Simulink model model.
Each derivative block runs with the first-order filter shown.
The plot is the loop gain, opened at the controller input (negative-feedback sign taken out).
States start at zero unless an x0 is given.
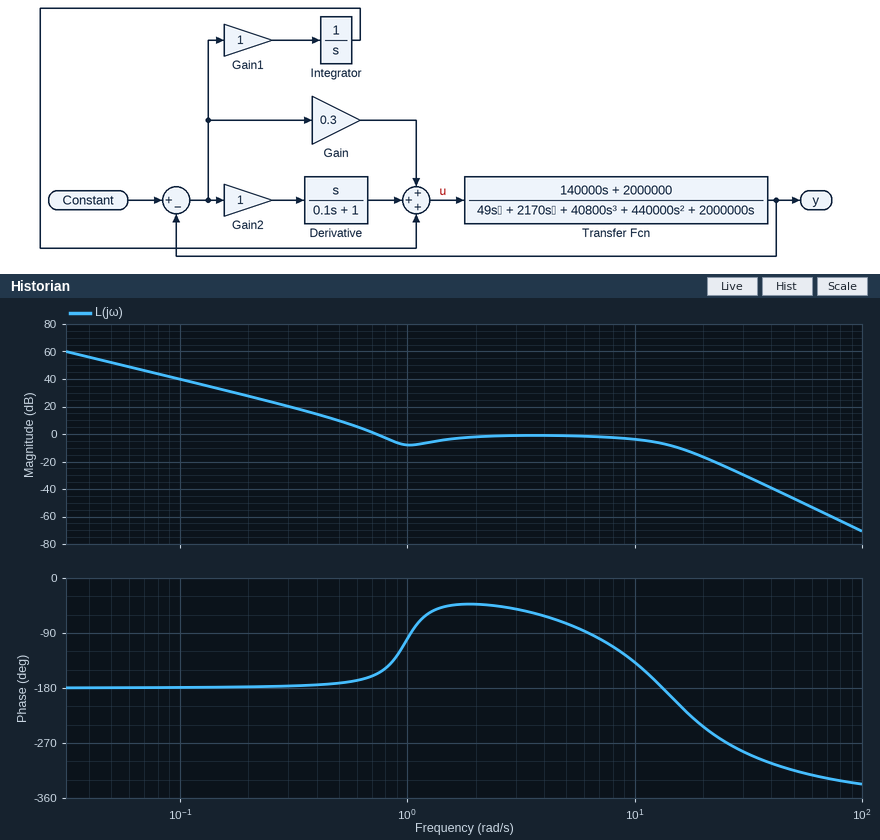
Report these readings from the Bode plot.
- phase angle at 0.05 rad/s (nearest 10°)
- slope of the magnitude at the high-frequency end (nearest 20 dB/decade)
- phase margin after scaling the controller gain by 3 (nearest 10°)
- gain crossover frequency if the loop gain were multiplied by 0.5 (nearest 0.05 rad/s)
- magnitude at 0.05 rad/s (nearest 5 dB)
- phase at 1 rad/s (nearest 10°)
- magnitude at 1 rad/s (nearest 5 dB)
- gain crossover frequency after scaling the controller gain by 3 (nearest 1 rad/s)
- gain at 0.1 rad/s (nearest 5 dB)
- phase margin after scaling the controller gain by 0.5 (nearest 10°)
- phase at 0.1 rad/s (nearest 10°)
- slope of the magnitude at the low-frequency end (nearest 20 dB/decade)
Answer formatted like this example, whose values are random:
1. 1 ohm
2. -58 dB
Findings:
1. -180°
2. -80 dB/decade
3. -20°
4. 0.60 rad/s
5. 50 dB
6. -100°
7. -10 dB
8. 15 rad/s
9. 40 dB
10. 10°
11. -180°
12. -40 dB/decade
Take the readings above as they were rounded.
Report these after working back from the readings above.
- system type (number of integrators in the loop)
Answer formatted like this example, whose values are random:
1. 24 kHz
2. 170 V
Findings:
1. 2
